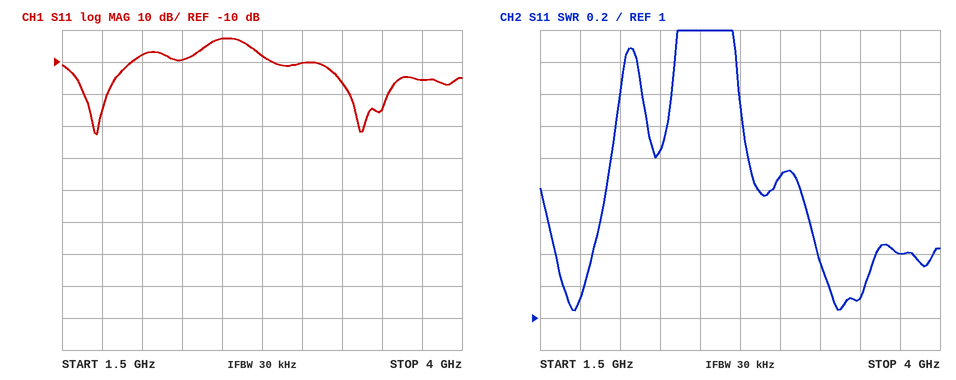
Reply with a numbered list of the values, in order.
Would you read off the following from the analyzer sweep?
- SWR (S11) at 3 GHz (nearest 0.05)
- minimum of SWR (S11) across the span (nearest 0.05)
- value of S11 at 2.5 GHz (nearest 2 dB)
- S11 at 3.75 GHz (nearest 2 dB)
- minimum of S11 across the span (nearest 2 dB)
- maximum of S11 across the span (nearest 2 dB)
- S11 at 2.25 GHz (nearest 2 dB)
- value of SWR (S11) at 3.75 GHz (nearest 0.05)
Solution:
1. 1.90
2. 1.05
3. -2 dB
4. -16 dB
5. -32 dB
6. -2 dB
7. -10 dB
8. 1.40
